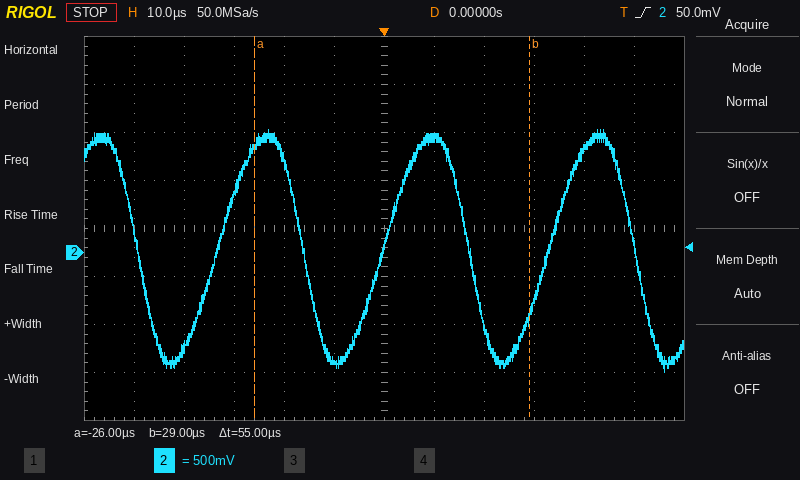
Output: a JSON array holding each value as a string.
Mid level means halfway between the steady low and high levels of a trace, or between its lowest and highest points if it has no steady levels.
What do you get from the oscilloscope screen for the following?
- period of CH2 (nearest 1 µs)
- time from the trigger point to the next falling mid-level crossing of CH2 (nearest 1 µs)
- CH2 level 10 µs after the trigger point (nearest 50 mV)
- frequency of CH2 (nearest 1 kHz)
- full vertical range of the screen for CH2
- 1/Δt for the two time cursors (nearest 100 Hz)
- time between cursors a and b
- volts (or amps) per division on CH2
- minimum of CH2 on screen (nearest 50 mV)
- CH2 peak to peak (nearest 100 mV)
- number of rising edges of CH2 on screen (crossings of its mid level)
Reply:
["33 µs", "17 µs", "1.20 V", "30 kHz", "4 V", "18.2 kHz", "55 µs", "500 mV", "-1.25 V", "2.50 V", "3"]
